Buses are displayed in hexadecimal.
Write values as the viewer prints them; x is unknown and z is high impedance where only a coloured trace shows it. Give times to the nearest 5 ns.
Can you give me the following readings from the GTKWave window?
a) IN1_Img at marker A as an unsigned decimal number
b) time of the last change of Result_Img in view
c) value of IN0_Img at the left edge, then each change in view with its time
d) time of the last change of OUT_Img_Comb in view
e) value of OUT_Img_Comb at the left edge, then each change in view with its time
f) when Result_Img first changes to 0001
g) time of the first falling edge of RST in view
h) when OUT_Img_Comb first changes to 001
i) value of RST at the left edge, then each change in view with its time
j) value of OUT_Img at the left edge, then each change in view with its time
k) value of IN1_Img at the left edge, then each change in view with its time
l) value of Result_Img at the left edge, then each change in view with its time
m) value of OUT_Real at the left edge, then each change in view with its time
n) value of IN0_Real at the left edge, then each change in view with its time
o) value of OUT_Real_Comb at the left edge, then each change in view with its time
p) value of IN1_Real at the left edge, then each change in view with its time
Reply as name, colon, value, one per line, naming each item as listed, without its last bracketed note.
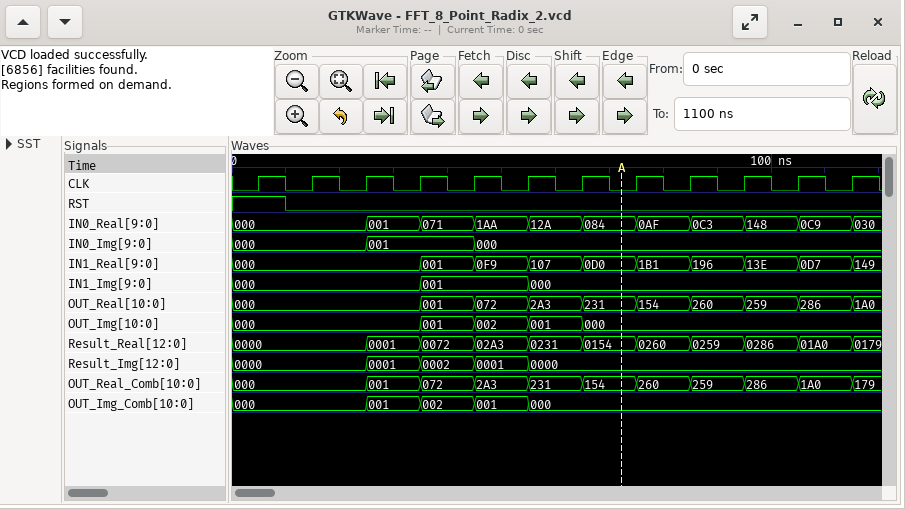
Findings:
IN1_Img at marker A as an unsigned decimal number: 0
time of the last change of Result_Img in view: 55 ns
value of IN0_Img at the left edge, then each change in view with its time: 000, 001 at 25 ns, 000 at 45 ns
time of the last change of OUT_Img_Comb in view: 55 ns
value of OUT_Img_Comb at the left edge, then each change in view with its time: 000, 001 at 25 ns, 002 at 35 ns, 001 at 45 ns, 000 at 55 ns
when Result_Img first changes to 0001: 25 ns
time of the first falling edge of RST in view: 10 ns
when OUT_Img_Comb first changes to 001: 25 ns
value of RST at the left edge, then each change in view with its time: 1, 0 at 10 ns
value of OUT_Img at the left edge, then each change in view with its time: 000, 001 at 35 ns, 002 at 45 ns, 001 at 55 ns, 000 at 65 ns
value of IN1_Img at the left edge, then each change in view with its time: 000, 001 at 35 ns, 000 at 55 ns
value of Result_Img at the left edge, then each change in view with its time: 0000, 0001 at 25 ns, 0002 at 35 ns, 0001 at 45 ns, 0000 at 55 ns
value of OUT_Real at the left edge, then each change in view with its time: 000, 001 at 35 ns, 072 at 45 ns, 2A3 at 55 ns, 231 at 65 ns, 154 at 75 ns, 260 at 85 ns, 259 at 95 ns, 286 at 105 ns, 1A0 at 115 ns
value of IN0_Real at the left edge, then each change in view with its time: 000, 001 at 25 ns, 071 at 35 ns, 1AA at 45 ns, 12A at 55 ns, 084 at 65 ns, 0AF at 75 ns, 0C3 at 85 ns, 148 at 95 ns, 0C9 at 105 ns, 030 at 115 ns
value of OUT_Real_Comb at the left edge, then each change in view with its time: 000, 001 at 25 ns, 072 at 35 ns, 2A3 at 45 ns, 231 at 55 ns, 154 at 65 ns, 260 at 75 ns, 259 at 85 ns, 286 at 95 ns, 1A0 at 105 ns, 179 at 115 ns
value of IN1_Real at the left edge, then each change in view with its time: 000, 001 at 35 ns, 0F9 at 45 ns, 107 at 55 ns, 0D0 at 65 ns, 1B1 at 75 ns, 196 at 85 ns, 13E at 95 ns, 0D7 at 105 ns, 149 at 115 ns
